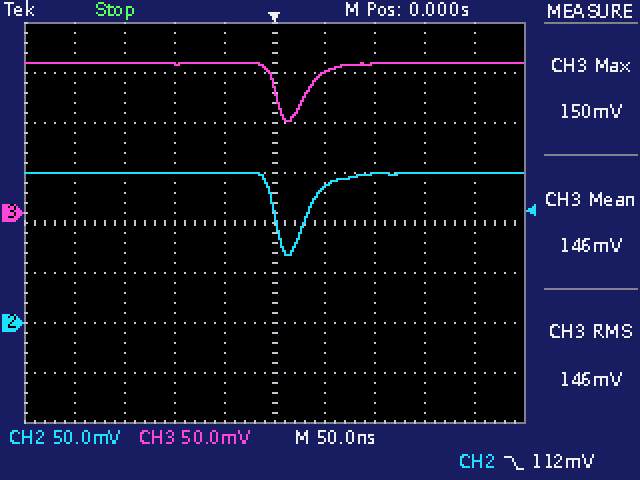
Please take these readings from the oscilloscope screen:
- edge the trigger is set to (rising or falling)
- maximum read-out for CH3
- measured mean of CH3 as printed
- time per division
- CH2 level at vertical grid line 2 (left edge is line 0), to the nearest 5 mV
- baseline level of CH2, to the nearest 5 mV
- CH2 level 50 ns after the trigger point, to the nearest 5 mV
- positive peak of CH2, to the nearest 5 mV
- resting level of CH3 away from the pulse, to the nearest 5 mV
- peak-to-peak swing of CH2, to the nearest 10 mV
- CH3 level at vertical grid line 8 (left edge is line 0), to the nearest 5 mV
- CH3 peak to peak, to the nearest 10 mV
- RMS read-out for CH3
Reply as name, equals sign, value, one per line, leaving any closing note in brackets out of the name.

edge the trigger is set to = falling
maximum read-out for CH3 = 150 mV
measured mean of CH3 as printed = 146 mV
time per division = 50 ns
CH2 level at vertical grid line 2 (left edge is line 0), to the nearest 5 mV = 150 mV
baseline level of CH2, to the nearest 5 mV = 150 mV
CH2 level 50 ns after the trigger point, to the nearest 5 mV = 135 mV
positive peak of CH2, to the nearest 5 mV = 150 mV
resting level of CH3 away from the pulse, to the nearest 5 mV = 150 mV
peak-to-peak swing of CH2, to the nearest 10 mV = 80 mV
CH3 level at vertical grid line 8 (left edge is line 0), to the nearest 5 mV = 150 mV
CH3 peak to peak, to the nearest 10 mV = 60 mV
RMS read-out for CH3 = 146 mV
